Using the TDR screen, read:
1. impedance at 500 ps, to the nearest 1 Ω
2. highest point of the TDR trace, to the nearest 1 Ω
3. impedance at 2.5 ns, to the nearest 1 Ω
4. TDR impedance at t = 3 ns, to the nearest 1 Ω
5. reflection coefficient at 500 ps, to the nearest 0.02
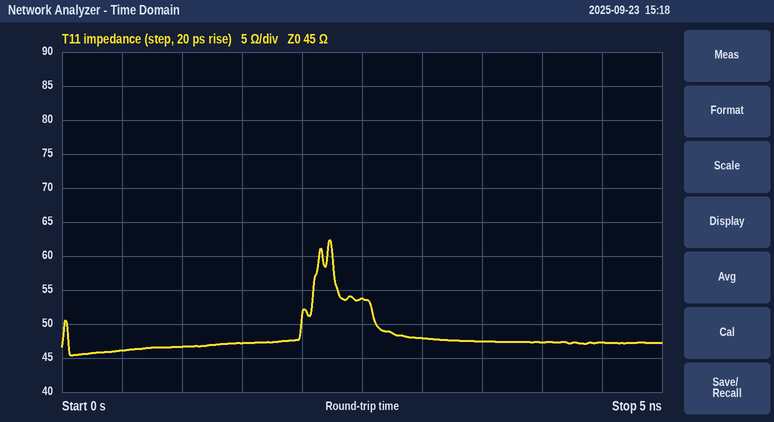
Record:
46 Ω
62 Ω
54 Ω
48 Ω
+0.02
